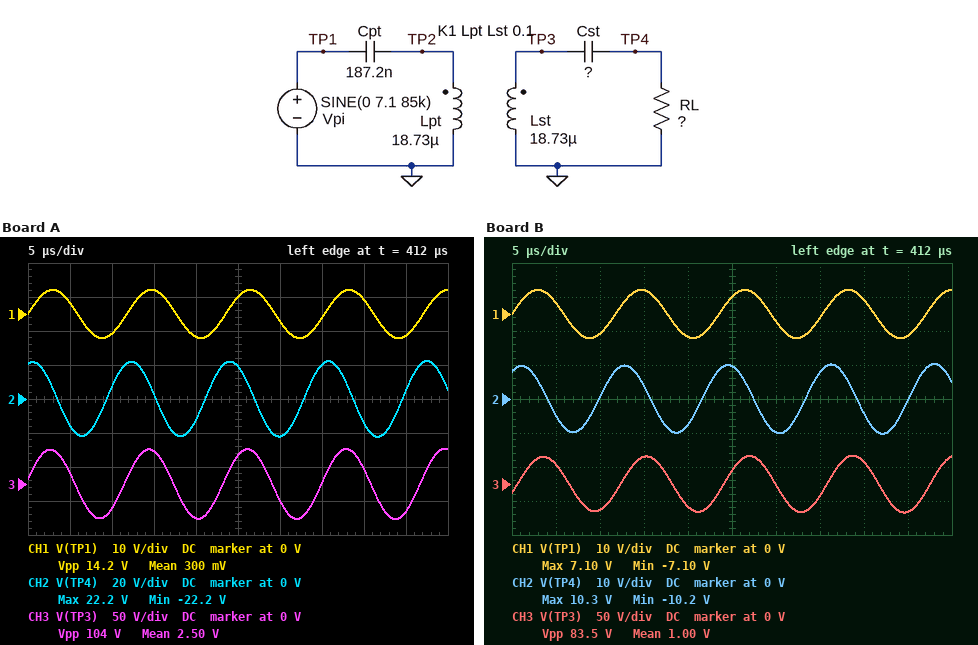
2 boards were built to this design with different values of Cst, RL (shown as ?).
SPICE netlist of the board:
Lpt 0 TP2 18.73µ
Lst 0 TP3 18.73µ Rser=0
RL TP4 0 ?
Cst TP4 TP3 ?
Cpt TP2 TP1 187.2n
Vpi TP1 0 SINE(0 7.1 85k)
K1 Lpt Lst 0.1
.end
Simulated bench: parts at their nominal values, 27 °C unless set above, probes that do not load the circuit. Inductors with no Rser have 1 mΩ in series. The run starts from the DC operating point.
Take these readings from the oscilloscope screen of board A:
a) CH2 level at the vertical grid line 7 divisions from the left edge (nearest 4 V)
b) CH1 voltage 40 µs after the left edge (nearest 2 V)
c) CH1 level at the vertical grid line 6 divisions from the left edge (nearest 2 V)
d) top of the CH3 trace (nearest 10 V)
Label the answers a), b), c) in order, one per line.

a) 20 V
b) 4 V
c) -2 V
d) 50 V
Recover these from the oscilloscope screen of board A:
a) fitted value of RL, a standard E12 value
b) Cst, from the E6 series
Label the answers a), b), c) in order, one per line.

a) 2.7 Ω
b) 330 nF
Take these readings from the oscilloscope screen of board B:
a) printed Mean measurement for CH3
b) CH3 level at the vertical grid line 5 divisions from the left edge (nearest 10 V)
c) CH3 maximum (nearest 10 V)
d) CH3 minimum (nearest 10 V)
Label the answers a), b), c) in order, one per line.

a) 1.00 V
b) 20 V
c) 40 V
d) -40 V
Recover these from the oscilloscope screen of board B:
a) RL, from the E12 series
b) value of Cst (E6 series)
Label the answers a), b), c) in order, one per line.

a) 1 Ω
b) 470 nF
